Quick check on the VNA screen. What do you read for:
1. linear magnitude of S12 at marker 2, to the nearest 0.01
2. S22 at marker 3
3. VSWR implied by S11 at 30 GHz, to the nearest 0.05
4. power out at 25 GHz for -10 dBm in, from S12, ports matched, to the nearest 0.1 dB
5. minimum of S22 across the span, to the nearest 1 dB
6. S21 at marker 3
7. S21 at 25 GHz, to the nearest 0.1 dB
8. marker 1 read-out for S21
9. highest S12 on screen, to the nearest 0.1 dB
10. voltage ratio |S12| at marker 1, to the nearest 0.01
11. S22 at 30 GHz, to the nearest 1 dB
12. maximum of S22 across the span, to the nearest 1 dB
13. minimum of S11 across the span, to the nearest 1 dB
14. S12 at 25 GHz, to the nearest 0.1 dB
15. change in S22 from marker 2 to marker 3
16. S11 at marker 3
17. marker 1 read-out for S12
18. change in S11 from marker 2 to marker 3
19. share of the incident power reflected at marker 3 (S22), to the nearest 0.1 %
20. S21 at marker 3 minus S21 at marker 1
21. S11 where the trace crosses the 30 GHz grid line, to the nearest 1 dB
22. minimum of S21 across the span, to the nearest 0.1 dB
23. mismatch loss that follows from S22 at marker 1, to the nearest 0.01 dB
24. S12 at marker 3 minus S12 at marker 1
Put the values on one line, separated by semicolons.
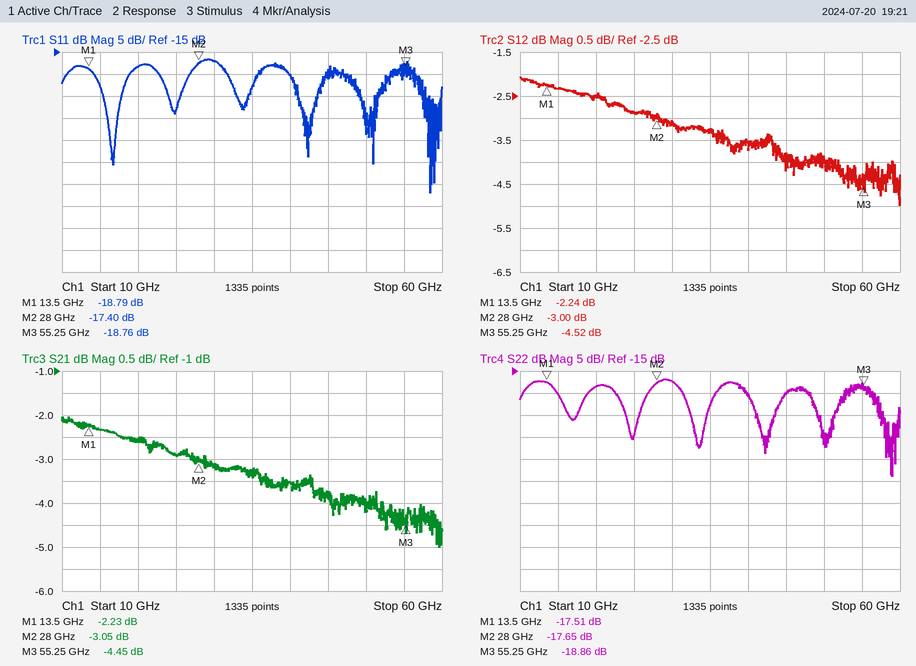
0.71; -18.86 dB; 1.35; -12.9 dBm; -39 dB; -4.45 dB; -2.9 dB; -2.23 dB; -2.1 dB; 0.77; -17 dB; -17 dB; -47 dB; -2.9 dB; -1.21 dB; -18.76 dB; -2.24 dB; -1.36 dB; 1.3 %; -2.22 dB; -17 dB; -5.0 dB; 0.08 dB; -2.28 dB
